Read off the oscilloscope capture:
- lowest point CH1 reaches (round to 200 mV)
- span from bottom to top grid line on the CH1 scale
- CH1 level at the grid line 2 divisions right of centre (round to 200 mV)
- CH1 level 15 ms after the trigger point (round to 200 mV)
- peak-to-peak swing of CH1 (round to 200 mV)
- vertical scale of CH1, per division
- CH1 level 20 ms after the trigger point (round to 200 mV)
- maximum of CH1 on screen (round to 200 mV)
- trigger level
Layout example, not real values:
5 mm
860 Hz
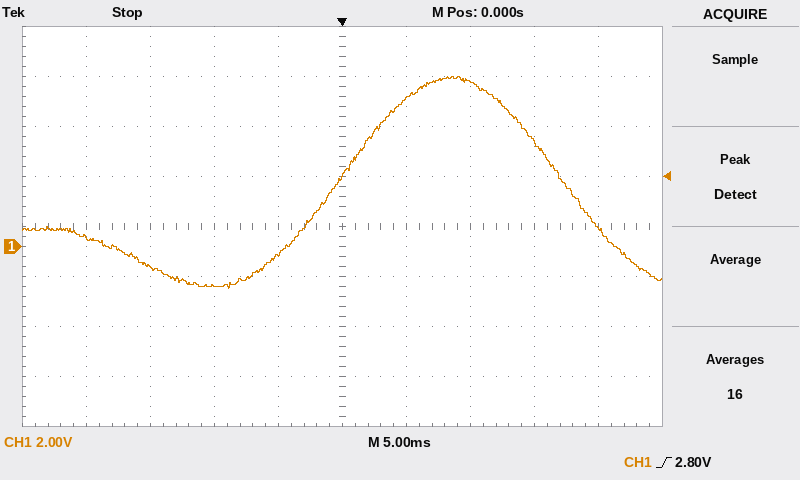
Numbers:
-1.6 V
16 V
6.6 V
4.2 V
8.4 V
2 V
800 mV
6.8 V
2.80 V
